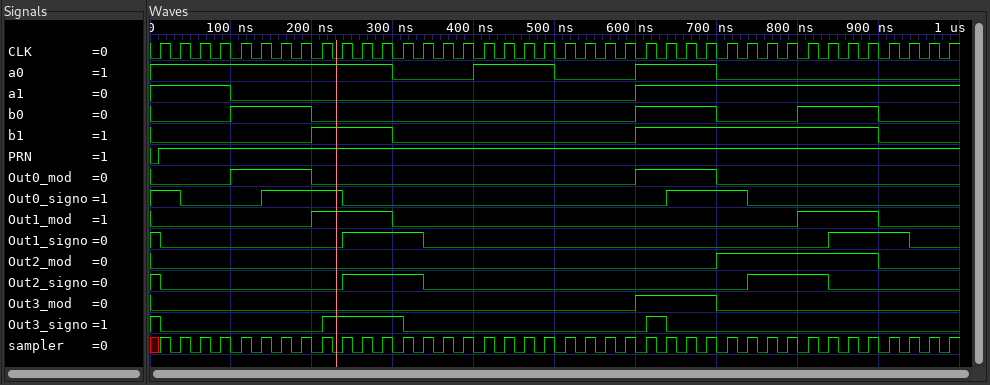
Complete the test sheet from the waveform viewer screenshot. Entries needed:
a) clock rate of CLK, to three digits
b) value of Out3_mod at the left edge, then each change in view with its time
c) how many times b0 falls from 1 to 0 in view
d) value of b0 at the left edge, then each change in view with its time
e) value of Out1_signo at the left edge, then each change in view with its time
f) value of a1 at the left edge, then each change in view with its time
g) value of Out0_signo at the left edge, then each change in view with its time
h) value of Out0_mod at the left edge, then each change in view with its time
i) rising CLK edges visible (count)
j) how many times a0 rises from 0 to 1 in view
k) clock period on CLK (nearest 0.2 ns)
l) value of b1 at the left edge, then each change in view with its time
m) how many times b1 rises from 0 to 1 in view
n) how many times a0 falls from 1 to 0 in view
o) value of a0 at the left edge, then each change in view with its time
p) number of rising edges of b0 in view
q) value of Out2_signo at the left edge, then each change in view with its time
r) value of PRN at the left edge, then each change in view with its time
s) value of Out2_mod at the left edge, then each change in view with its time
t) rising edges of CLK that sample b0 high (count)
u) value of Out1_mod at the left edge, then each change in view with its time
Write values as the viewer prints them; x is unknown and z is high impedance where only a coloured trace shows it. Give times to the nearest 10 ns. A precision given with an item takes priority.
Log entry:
40.0 MHz
0, 1 at 600 ns, 0 at 700 ns
3
0, 1 at 100 ns, 0 at 200 ns, 1 at 600 ns, 0 at 700 ns, 1 at 800 ns, 0 at 900 ns
1, 0 at 10 ns, 1 at 240 ns, 0 at 340 ns, 1 at 840 ns, 0 at 940 ns
1, 0 at 100 ns, 1 at 600 ns
1, 0 at 40 ns, 1 at 140 ns, 0 at 240 ns, 1 at 640 ns, 0 at 740 ns
0, 1 at 100 ns, 0 at 200 ns, 1 at 600 ns, 0 at 700 ns
40
2
25 ns
0, 1 at 200 ns, 0 at 300 ns, 1 at 600 ns, 0 at 900 ns
2
3
1, 0 at 300 ns, 1 at 400 ns, 0 at 500 ns, 1 at 600 ns, 0 at 700 ns
3
1, 0 at 10 ns, 1 at 240 ns, 0 at 340 ns, 1 at 740 ns, 0 at 840 ns
0, 1 at 10 ns
0, 1 at 700 ns, 0 at 900 ns
12
0, 1 at 200 ns, 0 at 300 ns, 1 at 800 ns, 0 at 900 ns
